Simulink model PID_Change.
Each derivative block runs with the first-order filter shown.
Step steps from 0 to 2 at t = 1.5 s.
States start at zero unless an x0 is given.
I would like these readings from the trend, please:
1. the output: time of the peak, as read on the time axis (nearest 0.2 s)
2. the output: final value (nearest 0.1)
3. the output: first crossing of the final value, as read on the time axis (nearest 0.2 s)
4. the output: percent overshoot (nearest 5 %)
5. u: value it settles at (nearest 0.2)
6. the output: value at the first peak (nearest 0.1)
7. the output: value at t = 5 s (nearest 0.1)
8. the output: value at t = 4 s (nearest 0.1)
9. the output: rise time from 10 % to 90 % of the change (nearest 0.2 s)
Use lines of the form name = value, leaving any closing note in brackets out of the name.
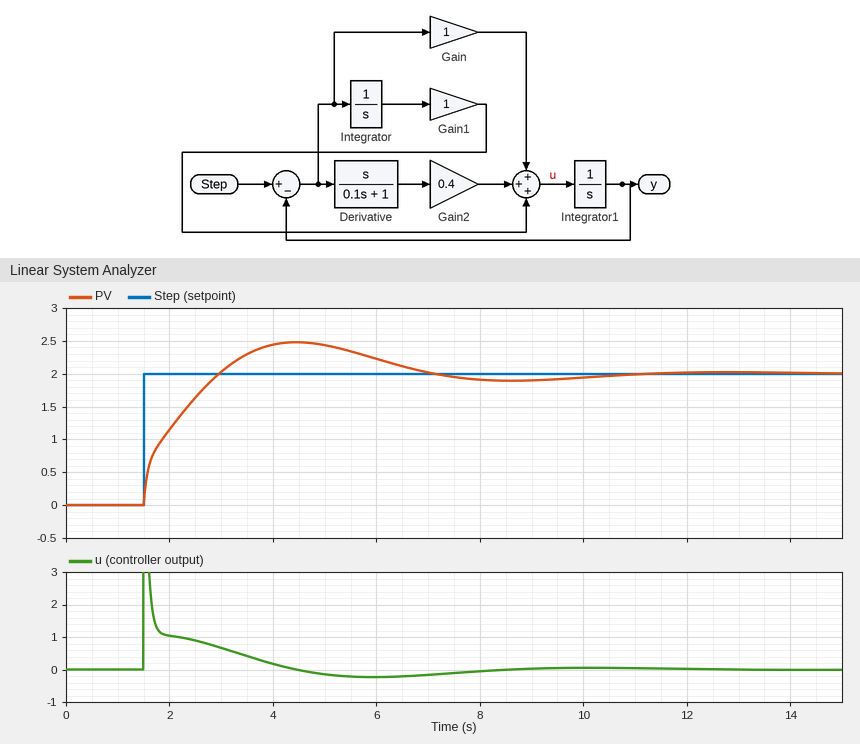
the output: time of the peak, as read on the time axis = 4.4 s
the output: final value = 2.0
the output: first crossing of the final value, as read on the time axis = 3.0 s
the output: percent overshoot = 25 %
u: value it settles at = 0.0
the output: value at the first peak = 2.5
the output: value at t = 5 s = 2.4
the output: value at t = 4 s = 2.4
the output: rise time from 10 % to 90 % of the change = 1.2 s
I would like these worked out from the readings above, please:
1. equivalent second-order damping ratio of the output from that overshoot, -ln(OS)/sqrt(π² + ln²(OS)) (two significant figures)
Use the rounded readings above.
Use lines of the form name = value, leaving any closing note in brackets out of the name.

equivalent second-order damping ratio of the output from that overshoot, -ln(OS)/sqrt(π² + ln²(OS)) = 0.40
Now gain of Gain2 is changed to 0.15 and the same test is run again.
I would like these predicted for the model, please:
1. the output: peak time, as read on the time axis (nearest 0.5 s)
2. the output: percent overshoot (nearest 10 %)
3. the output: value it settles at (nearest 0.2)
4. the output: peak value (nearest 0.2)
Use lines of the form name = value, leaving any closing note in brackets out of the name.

the output: peak time, as read on the time axis = 4.0 s
the output: percent overshoot = 30 %
the output: value it settles at = 2.0
the output: peak value = 2.6
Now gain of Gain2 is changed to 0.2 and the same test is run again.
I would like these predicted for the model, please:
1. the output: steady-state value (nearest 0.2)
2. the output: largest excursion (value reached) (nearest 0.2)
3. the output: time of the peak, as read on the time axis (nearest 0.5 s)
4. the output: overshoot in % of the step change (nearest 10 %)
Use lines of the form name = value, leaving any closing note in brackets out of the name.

the output: steady-state value = 2.0
the output: largest excursion (value reached) = 2.6
the output: time of the peak, as read on the time axis = 4.0 s
the output: overshoot in % of the step change = 30 %
